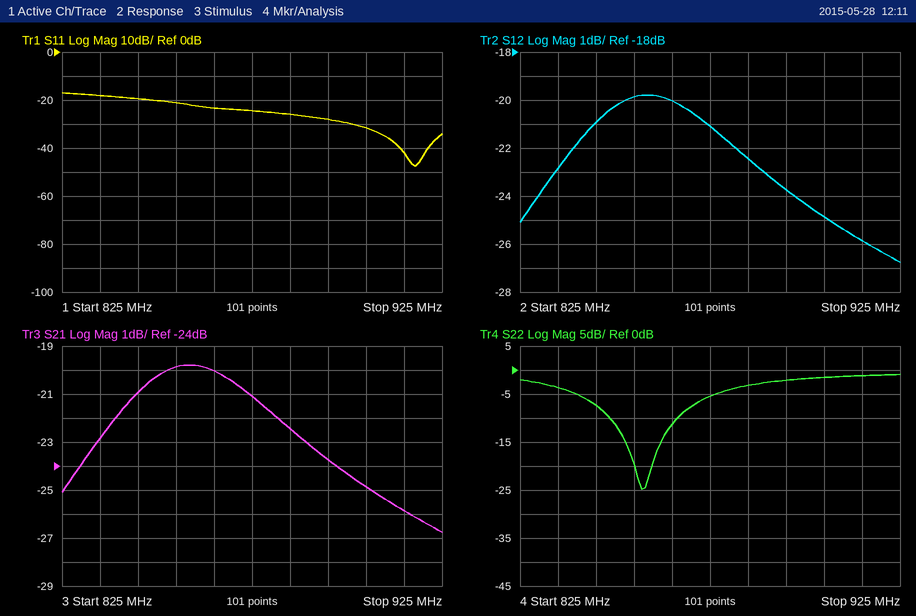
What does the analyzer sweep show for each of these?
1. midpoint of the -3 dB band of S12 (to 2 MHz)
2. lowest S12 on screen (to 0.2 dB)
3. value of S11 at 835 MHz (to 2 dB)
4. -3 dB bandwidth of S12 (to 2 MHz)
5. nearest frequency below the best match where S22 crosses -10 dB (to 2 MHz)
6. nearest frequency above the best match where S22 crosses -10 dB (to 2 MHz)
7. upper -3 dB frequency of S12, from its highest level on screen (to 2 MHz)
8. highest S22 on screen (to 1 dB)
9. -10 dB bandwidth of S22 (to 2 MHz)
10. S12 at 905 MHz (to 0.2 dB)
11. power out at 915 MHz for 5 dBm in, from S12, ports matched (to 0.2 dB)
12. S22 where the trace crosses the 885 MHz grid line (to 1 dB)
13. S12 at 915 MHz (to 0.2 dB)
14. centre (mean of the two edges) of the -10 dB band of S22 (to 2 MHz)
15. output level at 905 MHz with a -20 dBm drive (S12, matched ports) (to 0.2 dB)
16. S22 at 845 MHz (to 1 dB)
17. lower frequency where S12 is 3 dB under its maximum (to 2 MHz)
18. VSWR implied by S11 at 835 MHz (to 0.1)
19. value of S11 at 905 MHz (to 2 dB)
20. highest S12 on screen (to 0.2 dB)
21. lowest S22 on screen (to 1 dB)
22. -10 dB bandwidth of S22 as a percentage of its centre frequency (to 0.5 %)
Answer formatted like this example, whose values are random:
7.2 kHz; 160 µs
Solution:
862 MHz; -26.8 dB; -18 dB; 52 MHz; 848 MHz; 866 MHz; 888 MHz; -1 dB; 18 MHz; -24.8 dB; -20.8 dBm; -3 dB; -25.8 dB; 858 MHz; -44.8 dBm; -7 dB; 836 MHz; 1.3; -32 dB; -19.8 dB; -25 dB; 2.0 %
